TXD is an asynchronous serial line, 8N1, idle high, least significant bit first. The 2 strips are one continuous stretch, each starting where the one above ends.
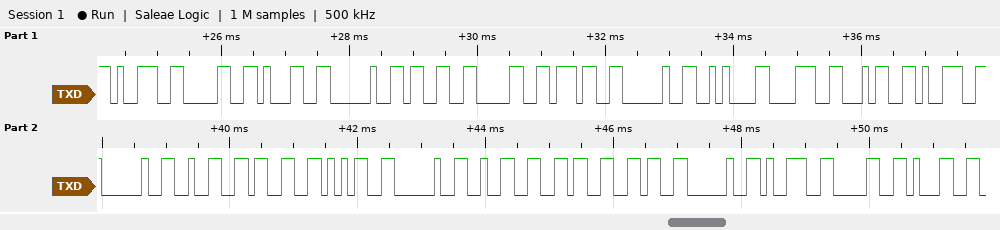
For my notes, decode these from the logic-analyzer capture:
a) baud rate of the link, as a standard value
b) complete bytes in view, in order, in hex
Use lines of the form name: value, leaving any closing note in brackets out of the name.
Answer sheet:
baud rate of the link, as a standard value: 9600 baud
complete bytes in view, in order, in hex: 0x39 0x30 0x31 0x20 0x33 0x30 0x37 0x20 0x0A 0x38 0x34 0x39 0x20 0x32 0x33 0x35 0x20 0x32 0x36 0x36 0x20 0x39 0x30 0x31
